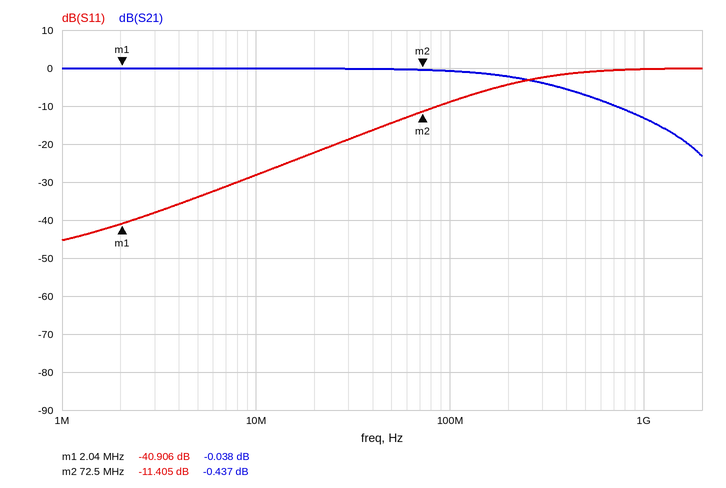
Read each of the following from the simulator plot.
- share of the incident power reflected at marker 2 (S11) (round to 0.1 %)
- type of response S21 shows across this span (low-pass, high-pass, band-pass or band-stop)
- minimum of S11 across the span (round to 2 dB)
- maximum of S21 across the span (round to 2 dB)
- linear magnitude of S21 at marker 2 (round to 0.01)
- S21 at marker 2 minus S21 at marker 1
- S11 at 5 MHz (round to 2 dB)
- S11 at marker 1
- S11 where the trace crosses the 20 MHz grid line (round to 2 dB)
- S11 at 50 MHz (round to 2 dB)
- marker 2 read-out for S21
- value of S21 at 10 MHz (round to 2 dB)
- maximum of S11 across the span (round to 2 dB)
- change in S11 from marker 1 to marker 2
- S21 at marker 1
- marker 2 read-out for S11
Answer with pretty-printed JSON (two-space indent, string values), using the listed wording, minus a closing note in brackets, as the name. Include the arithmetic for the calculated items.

{
  "share of the incident power reflected at marker 2 (S11)": "10^(-11.405/10) ≈ 7.2 %",
  "type of response S21 shows across this span": "low-pass",
  "minimum of S11 across the span": "-46 dB",
  "maximum of S21 across the span": "0 dB",
  "linear magnitude of S21 at marker 2": "10^(-0.437/20) ≈ 0.95",
  "S21 at marker 2 minus S21 at marker 1": "-0.437 − (-0.038) = -0.399 dB",
  "S11 at 5 MHz": "-34 dB",
  "S11 at marker 1": "-40.906 dB",
  "S11 where the trace crosses the 20 MHz grid line": "-22 dB",
  "S11 at 50 MHz": "-14 dB",
  "marker 2 read-out for S21": "-0.437 dB",
  "value of S21 at 10 MHz": "0 dB",
  "maximum of S11 across the span": "0 dB",
  "change in S11 from marker 1 to marker 2": "-11.405 − (-40.906) = 29.501 dB",
  "S21 at marker 1": "-0.038 dB",
  "marker 2 read-out for S11": "-11.405 dB"
}
